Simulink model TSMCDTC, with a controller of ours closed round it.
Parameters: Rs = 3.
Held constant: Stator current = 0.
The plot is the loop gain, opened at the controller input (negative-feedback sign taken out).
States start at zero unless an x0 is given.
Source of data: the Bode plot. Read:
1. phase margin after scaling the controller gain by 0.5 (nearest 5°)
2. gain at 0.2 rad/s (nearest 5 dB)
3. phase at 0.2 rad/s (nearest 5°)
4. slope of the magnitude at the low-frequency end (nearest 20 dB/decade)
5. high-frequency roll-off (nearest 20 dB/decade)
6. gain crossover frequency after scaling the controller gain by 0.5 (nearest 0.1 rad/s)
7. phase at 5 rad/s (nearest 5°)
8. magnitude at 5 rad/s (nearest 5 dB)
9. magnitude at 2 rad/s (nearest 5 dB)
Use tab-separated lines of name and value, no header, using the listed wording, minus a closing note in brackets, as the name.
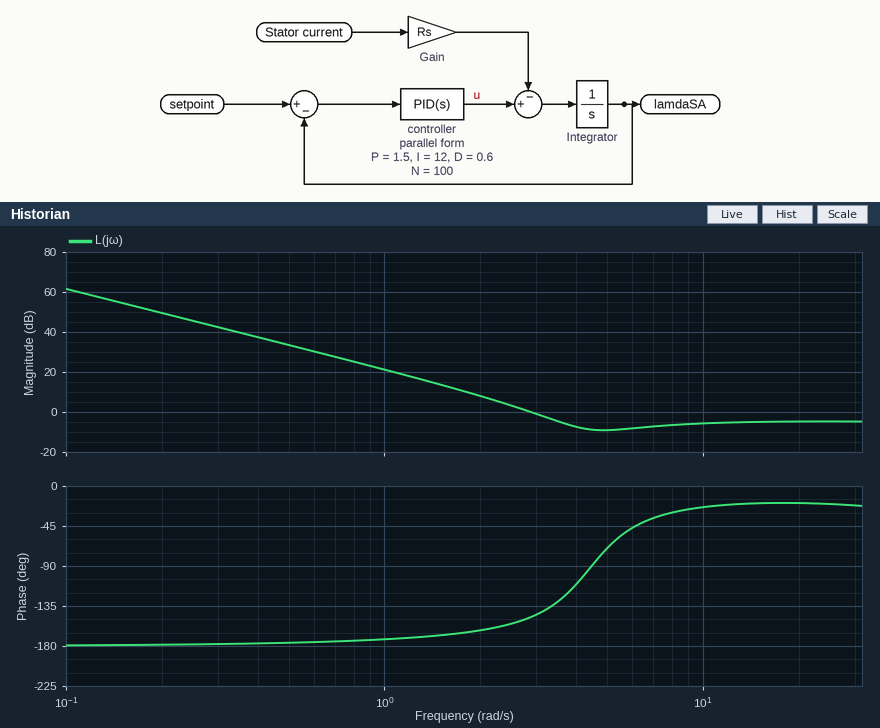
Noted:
phase margin after scaling the controller gain by 0.5	20°
gain at 0.2 rad/s	50 dB
phase at 0.2 rad/s	-180°
slope of the magnitude at the low-frequency end	-40 dB/decade
high-frequency roll-off	0 dB/decade
gain crossover frequency after scaling the controller gain by 0.5	2.2 rad/s
phase at 5 rad/s	-70°
magnitude at 5 rad/s	-10 dB
magnitude at 2 rad/s	10 dB
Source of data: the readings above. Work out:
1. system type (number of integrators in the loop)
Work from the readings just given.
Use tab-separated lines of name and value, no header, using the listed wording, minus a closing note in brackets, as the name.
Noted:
system type	2
